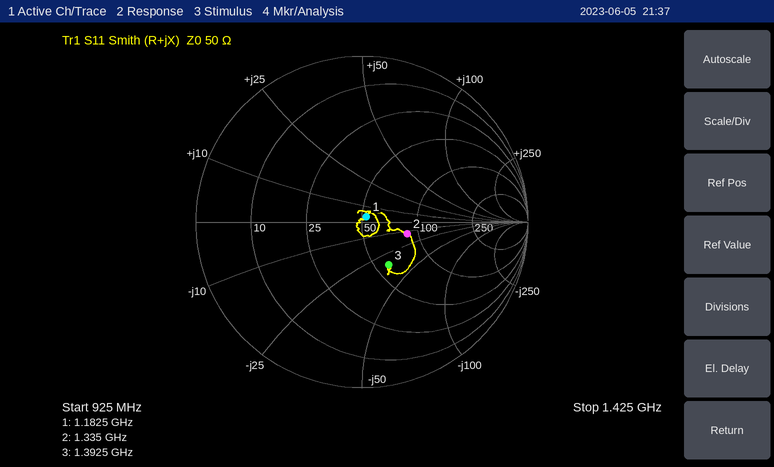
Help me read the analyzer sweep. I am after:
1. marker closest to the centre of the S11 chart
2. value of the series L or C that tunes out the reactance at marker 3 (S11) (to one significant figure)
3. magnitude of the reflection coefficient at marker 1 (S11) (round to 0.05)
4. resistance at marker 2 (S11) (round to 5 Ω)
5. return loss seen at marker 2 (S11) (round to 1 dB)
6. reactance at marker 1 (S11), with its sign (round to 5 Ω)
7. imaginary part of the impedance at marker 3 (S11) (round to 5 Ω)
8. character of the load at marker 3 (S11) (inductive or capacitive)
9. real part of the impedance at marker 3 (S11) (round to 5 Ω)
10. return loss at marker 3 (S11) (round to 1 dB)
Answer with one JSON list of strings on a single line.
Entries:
["marker 1", "4 nH", "0.05", "85 Ω", "11 dB", "+5 Ω", "-35 Ω", "capacitive", "60 Ω", "10 dB"]
